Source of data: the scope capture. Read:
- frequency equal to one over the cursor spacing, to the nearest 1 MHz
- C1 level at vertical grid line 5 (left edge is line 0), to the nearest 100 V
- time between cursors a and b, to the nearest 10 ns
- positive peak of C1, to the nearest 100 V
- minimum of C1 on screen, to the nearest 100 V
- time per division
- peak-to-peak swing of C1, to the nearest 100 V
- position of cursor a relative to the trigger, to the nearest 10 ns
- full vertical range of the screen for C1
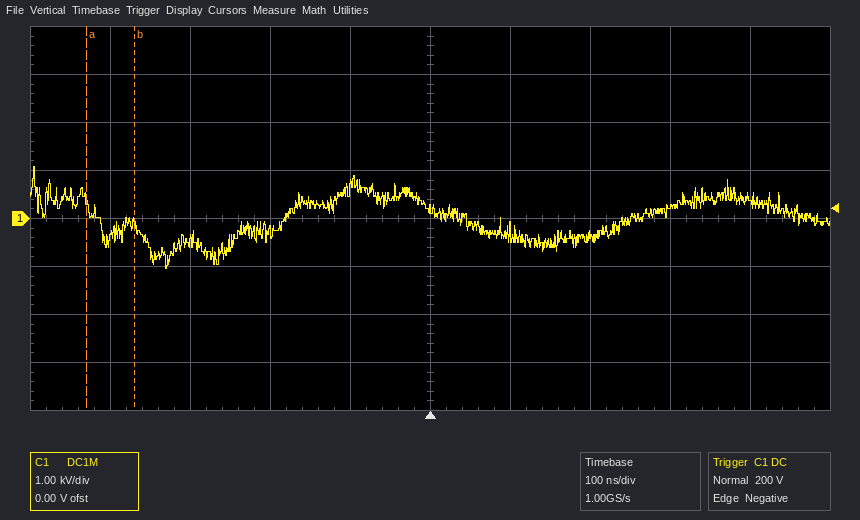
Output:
17 MHz
200 V
60 ns
1.1 kV
-1.0 kV
100 ns
2.1 kV
-430 ns
8 kV
